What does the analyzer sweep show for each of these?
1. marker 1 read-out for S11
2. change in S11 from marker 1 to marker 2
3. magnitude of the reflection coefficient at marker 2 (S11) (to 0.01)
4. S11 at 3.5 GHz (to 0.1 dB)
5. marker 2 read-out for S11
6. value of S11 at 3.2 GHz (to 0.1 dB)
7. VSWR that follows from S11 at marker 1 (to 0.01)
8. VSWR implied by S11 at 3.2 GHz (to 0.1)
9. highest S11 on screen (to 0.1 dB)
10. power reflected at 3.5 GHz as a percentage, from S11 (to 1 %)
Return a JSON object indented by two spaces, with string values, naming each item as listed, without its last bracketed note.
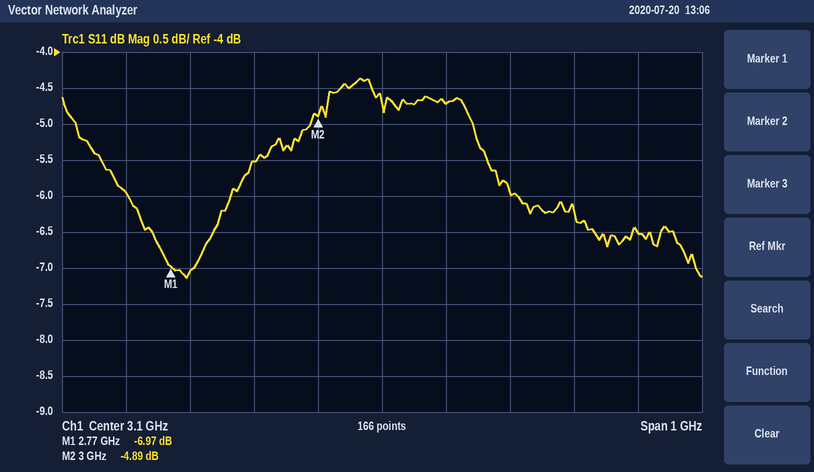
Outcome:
{
  "marker 1 read-out for S11": "-6.97 dB",
  "change in S11 from marker 1 to marker 2": "2.08 dB",
  "magnitude of the reflection coefficient at marker 2 (S11)": "0.57",
  "S11 at 3.5 GHz": "-6.5 dB",
  "marker 2 read-out for S11": "-4.89 dB",
  "value of S11 at 3.2 GHz": "-4.7 dB",
  "VSWR that follows from S11 at marker 1": "2.62",
  "VSWR implied by S11 at 3.2 GHz": "3.8",
  "highest S11 on screen": "-4.4 dB",
  "power reflected at 3.5 GHz as a percentage, from S11": "22 %"
}
